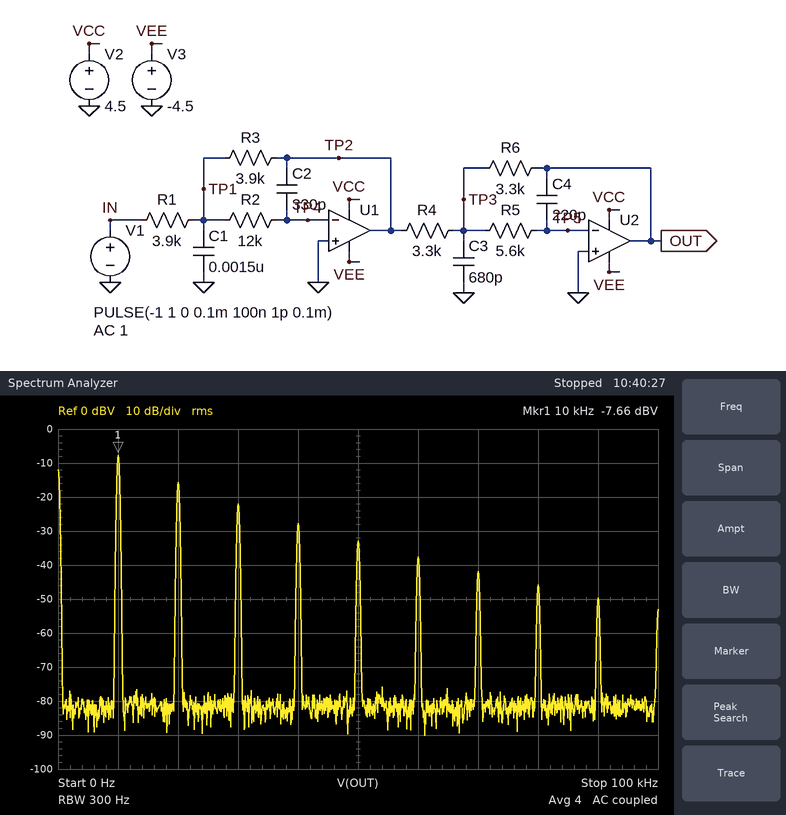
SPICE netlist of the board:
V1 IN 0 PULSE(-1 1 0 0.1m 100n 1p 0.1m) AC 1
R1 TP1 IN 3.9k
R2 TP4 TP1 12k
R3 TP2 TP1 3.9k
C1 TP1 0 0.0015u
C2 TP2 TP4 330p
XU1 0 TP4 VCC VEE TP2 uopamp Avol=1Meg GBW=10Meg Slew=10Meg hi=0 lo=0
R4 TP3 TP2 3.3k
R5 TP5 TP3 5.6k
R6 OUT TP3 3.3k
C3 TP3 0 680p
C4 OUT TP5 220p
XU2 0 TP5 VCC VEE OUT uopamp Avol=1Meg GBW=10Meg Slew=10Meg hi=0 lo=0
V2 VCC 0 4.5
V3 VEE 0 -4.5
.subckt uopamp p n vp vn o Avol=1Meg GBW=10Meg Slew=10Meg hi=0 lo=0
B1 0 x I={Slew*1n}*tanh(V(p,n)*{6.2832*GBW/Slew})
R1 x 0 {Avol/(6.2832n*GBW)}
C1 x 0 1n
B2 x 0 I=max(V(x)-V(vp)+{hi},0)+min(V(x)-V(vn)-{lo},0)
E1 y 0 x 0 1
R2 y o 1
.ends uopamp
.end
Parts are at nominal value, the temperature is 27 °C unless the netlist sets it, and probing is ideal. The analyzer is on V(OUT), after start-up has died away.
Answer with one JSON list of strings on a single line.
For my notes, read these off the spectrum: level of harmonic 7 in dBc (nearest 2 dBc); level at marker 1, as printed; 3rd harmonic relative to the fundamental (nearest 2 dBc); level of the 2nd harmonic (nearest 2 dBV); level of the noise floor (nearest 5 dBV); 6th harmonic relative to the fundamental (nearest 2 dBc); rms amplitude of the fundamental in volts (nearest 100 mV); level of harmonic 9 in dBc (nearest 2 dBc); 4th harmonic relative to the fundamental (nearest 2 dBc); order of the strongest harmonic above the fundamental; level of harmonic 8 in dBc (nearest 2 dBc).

["-34 dBc", "-7.66 dBV", "-14 dBc", "-16 dBV", "-80 dBV", "-30 dBc", "400 mV", "-42 dBc", "-20 dBc", "2", "-38 dBc"]
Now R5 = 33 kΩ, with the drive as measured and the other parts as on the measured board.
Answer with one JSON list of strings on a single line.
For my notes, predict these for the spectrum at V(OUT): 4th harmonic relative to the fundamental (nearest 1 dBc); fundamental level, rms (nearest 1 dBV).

["-28 dBc", "-10 dBV"]
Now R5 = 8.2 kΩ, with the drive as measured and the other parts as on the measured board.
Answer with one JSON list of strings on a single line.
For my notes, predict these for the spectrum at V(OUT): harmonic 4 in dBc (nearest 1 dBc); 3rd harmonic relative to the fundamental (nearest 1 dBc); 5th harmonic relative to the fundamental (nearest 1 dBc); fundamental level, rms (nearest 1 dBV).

["-21 dBc", "-15 dBc", "-27 dBc", "-8 dBV"]
